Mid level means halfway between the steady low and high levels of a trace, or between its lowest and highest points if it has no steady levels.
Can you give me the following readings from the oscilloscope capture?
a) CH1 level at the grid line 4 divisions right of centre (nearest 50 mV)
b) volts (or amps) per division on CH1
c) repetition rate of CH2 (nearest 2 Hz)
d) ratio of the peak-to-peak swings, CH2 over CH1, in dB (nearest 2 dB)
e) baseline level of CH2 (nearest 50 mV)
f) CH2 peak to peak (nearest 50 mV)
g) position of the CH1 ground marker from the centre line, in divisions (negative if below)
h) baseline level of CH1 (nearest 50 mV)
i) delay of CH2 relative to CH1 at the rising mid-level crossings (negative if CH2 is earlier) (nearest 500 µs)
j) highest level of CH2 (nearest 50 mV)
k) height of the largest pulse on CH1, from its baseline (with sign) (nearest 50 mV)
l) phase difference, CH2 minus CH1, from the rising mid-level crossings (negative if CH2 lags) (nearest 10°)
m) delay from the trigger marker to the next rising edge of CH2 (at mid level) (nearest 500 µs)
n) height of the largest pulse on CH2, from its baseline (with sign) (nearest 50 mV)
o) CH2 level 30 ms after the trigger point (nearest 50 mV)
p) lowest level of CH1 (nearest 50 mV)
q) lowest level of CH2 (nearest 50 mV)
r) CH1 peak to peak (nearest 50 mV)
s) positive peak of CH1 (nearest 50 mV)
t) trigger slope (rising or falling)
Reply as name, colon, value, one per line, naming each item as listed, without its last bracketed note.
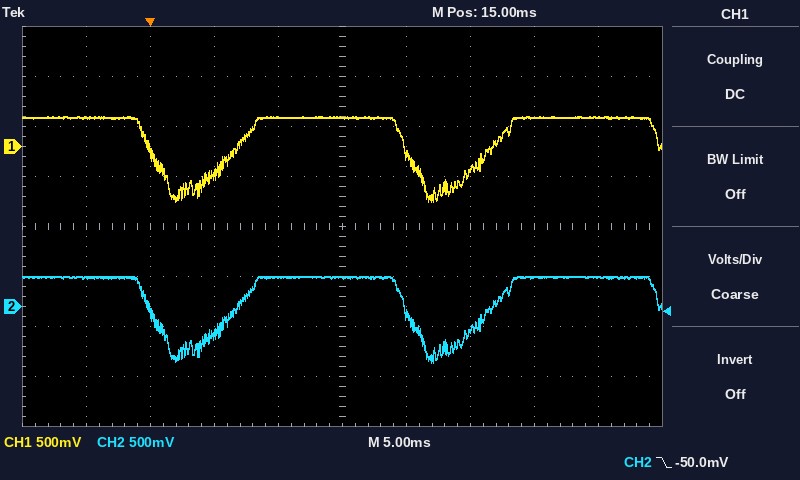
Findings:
CH1 level at the grid line 4 divisions right of centre: 300 mV
volts (or amps) per division on CH1: 500 mV
repetition rate of CH2: 50 Hz
ratio of the peak-to-peak swings, CH2 over CH1, in dB: 0 dB
baseline level of CH2: 300 mV
CH2 peak to peak: 850 mV
position of the CH1 ground marker from the centre line, in divisions: +1.6 div
baseline level of CH1: 300 mV
delay of CH2 relative to CH1 at the rising mid-level crossings (negative if CH2 is earlier): 0.0 ms
highest level of CH2: 300 mV
height of the largest pulse on CH1, from its baseline (with sign): -850 mV
phase difference, CH2 minus CH1, from the rising mid-level crossings (negative if CH2 lags): 0°
delay from the trigger marker to the next rising edge of CH2 (at mid level): 6.0 ms
height of the largest pulse on CH2, from its baseline (with sign): -850 mV
CH2 level 30 ms after the trigger point: 300 mV
lowest level of CH1: -550 mV
lowest level of CH2: -550 mV
CH1 peak to peak: 850 mV
positive peak of CH1: 300 mV
trigger slope: falling
